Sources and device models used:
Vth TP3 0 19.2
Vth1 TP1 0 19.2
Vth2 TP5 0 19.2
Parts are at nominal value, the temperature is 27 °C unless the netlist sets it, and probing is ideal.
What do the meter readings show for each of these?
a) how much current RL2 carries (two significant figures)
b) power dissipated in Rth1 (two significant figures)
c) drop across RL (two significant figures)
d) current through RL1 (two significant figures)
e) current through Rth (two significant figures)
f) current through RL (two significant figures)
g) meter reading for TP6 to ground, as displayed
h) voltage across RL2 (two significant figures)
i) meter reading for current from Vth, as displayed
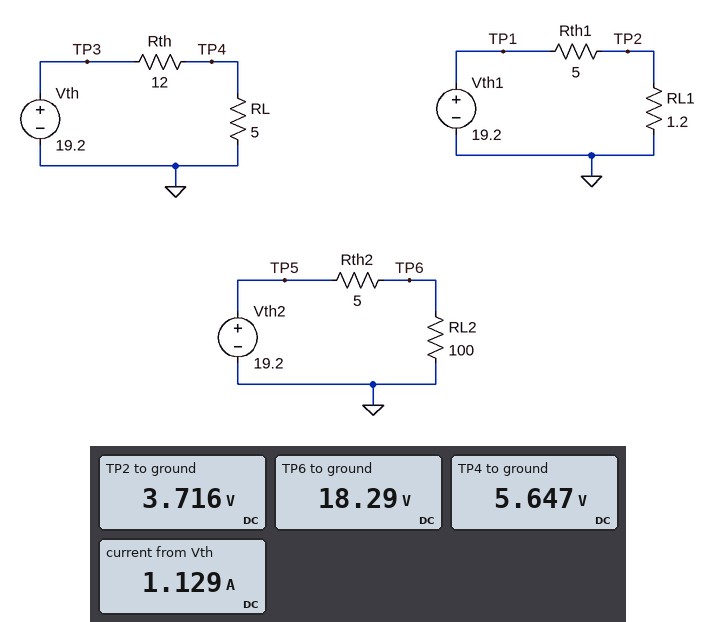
180 mA
48 W
5.6 V
3.1 A
1.1 A
1.1 A
18.29 V
18 V
1.129 A
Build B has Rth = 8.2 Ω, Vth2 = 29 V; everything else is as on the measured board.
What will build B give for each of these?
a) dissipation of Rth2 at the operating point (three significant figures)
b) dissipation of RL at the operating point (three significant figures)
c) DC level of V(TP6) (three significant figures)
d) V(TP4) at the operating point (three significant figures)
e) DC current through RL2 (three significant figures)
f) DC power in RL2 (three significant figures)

381 mW
10.6 W
27.6 V
7.27 V
276 mA
7.63 W
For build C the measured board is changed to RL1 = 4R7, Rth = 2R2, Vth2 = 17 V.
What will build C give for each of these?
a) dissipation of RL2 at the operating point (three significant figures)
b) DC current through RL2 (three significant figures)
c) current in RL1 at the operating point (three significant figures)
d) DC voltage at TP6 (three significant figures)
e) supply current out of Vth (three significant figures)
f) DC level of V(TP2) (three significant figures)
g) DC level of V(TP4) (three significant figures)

2.62 W
162 mA
1.98 A
16.2 V
2.67 A
9.30 V
13.3 V
